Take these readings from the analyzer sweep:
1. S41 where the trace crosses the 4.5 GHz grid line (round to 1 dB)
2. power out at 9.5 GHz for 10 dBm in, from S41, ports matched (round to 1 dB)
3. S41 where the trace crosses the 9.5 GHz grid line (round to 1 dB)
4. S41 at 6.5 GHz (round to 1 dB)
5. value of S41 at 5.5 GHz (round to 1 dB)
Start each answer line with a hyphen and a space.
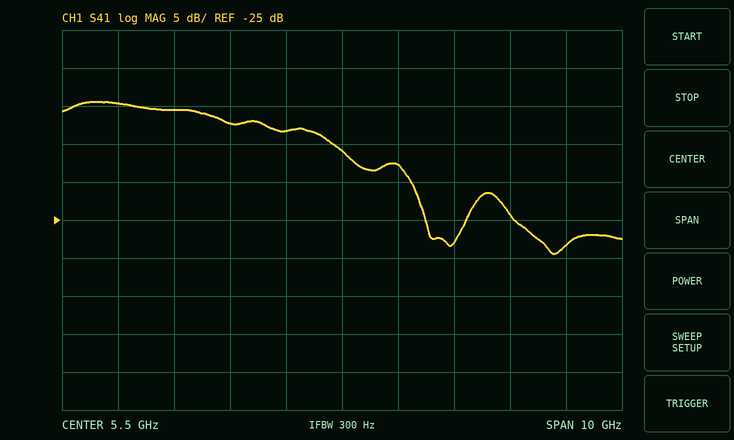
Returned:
- -13 dB
- -18 dBm
- -28 dB
- -18 dB
- -16 dB
